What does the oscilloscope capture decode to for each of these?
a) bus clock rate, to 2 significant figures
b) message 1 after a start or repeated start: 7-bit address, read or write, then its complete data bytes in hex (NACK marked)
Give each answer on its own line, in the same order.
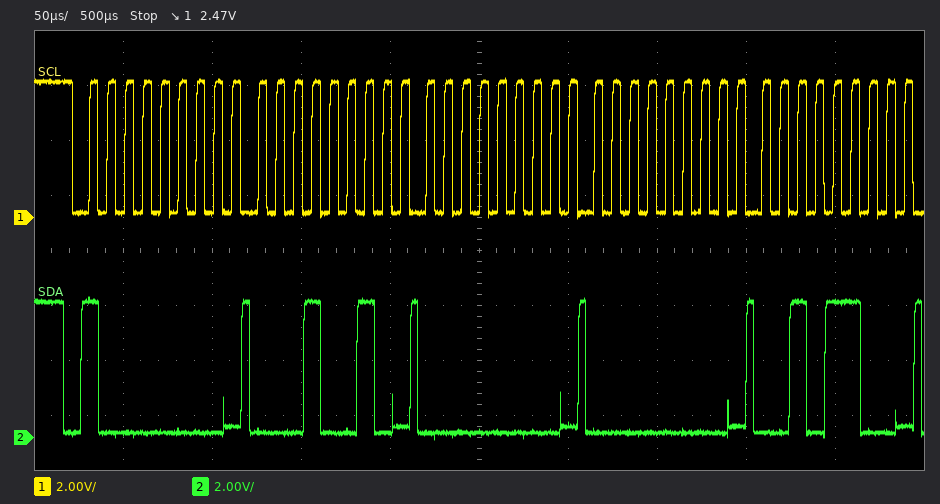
100 kHz
0x40 write: 12 00 00 2C
